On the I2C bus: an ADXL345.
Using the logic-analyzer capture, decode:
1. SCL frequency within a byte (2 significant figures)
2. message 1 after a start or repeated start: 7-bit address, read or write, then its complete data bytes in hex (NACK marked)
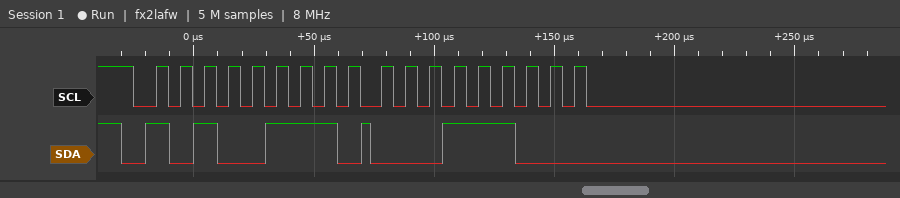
100 kHz
0x53 read: 1C
